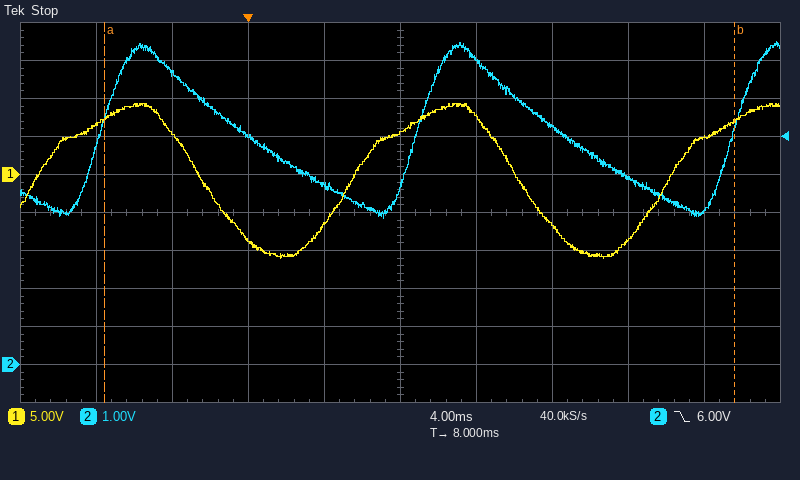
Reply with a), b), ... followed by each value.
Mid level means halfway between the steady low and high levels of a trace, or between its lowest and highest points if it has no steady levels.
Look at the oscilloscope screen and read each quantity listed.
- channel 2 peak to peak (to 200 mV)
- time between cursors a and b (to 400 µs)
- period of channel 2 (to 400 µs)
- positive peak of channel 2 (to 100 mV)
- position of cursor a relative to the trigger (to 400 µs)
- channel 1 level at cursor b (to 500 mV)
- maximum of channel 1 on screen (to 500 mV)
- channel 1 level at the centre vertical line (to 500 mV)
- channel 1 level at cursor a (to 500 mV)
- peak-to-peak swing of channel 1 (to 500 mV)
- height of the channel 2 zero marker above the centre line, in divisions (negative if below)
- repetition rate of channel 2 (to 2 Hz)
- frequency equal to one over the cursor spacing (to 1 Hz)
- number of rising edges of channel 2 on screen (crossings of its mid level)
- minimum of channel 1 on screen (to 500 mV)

a) 4.6 V
b) 33.2 ms
c) 16.8 ms
d) 8.5 V
e) -7.6 ms
f) 7.0 V
g) 9.5 V
h) 5.5 V
i) 7.5 V
j) 20.5 V
k) -4.0 div
l) 60 Hz
m) 30 Hz
n) 3
o) -11.0 V
